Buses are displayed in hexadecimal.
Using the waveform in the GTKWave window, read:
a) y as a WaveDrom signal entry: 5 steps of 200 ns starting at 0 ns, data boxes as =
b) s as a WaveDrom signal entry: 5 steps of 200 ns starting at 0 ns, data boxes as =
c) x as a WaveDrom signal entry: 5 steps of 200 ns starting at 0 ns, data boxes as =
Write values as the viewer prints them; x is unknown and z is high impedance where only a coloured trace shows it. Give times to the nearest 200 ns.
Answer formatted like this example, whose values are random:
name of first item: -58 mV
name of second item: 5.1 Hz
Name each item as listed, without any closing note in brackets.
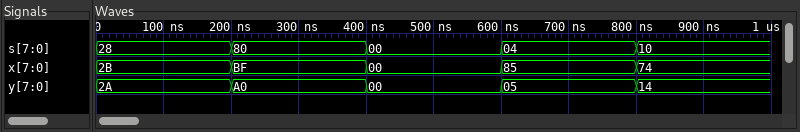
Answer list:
y as a WaveDrom signal entry: 5 steps of 200 ns starting at 0 ns, data boxes as =: {name: 'y', wave: '=====', data: '2A A0 00 05 14'}
s as a WaveDrom signal entry: 5 steps of 200 ns starting at 0 ns, data boxes as =: {name: 's', wave: '=====', data: '28 80 00 04 10'}
x as a WaveDrom signal entry: 5 steps of 200 ns starting at 0 ns, data boxes as =: {name: 'x', wave: '=====', data: '2B BF 00 85 74'}
